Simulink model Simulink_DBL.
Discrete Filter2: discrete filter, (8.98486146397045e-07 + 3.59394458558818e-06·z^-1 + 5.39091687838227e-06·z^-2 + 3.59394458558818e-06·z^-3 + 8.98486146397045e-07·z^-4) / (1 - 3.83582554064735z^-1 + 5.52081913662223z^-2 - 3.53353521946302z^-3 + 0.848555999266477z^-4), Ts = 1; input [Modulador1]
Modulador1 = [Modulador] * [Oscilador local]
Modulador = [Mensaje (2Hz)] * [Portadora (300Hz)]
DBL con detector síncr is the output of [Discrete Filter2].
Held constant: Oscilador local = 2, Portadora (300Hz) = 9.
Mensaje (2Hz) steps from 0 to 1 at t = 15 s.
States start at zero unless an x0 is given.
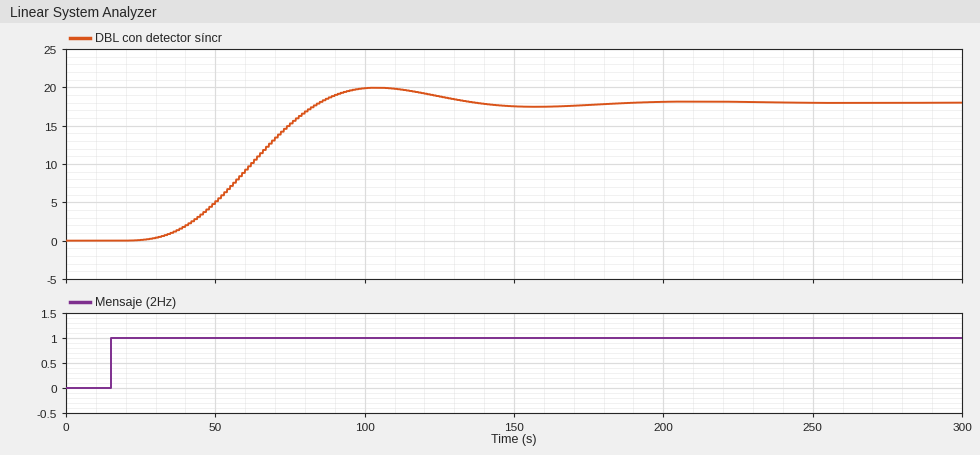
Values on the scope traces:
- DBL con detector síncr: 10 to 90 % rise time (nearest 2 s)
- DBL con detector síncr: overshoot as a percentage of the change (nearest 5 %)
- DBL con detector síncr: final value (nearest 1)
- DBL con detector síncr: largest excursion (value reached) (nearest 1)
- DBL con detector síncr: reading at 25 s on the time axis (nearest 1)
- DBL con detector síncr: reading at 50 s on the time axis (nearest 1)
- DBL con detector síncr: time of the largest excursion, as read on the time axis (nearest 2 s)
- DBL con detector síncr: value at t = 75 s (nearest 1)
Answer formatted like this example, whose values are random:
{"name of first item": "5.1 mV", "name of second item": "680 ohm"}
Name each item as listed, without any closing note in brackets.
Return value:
{"DBL con detector síncr: 10 to 90 % rise time": "38 s", "DBL con detector síncr: overshoot as a percentage of the change": "10 %", "DBL con detector síncr: final value": "18", "DBL con detector síncr: largest excursion (value reached)": "20", "DBL con detector síncr: reading at 25 s on the time axis": "0", "DBL con detector síncr: reading at 50 s on the time axis": "5", "DBL con detector síncr: time of the largest excursion, as read on the time axis": "104 s", "DBL con detector síncr: value at t = 75 s": "15"}
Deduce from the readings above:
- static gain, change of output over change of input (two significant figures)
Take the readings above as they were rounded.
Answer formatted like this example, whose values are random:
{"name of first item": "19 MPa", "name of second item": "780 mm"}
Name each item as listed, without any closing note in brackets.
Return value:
{"static gain, change of output over change of input": "18"}
